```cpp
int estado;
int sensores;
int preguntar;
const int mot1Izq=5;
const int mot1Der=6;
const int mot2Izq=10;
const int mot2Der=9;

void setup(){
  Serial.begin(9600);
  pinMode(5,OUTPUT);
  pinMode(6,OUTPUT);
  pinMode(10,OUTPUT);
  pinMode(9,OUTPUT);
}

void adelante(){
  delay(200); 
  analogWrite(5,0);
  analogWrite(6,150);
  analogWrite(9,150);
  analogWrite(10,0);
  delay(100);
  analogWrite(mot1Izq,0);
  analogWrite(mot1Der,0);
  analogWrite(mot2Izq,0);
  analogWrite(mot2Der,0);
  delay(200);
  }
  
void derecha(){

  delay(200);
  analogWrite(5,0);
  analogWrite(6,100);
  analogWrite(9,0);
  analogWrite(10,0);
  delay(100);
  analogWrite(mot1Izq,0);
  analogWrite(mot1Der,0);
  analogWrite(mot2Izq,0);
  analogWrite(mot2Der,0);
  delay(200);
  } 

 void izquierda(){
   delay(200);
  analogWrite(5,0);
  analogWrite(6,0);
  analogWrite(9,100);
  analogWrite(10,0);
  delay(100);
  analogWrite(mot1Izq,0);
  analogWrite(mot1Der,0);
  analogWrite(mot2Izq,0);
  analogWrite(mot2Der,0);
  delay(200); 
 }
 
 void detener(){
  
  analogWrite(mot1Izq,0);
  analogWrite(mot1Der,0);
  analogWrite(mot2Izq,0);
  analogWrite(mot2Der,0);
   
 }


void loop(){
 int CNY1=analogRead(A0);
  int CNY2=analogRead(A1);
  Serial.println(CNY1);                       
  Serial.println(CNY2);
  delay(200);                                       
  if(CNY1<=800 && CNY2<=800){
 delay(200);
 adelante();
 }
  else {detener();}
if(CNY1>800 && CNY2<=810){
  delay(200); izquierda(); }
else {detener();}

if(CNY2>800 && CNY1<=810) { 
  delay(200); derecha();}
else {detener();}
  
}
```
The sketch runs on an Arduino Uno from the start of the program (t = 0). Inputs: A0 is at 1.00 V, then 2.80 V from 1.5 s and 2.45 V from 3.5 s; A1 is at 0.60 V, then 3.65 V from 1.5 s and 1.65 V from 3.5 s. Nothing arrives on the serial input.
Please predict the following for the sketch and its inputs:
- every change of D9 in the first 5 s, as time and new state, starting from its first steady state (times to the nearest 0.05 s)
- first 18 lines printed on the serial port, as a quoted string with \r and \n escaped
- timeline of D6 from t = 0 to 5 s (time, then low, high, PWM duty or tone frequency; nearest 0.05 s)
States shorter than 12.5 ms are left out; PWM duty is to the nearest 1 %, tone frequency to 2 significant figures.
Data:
0 s low; 0.6 s PWM 59 %; 0.7 s low; 1.5 s PWM 59 %; 1.6 s low; 2.4 s PWM 59 %; 2.5 s low; 3.3 s PWM 59 %; 3.4 s low; 4.2 s PWM 59 %; 4.3 s low
"204\r\n122\r\n204\r\n122\r\n573\r\n747\r\n573\r\n747\r\n501\r\n337\r\n501\r\n337\r\n501\r\n337\r\n501\r\n337\r\n501\r\n337\r\n"
0 s low; 0.6 s PWM 59 %; 0.7 s low; 1.5 s PWM 59 %; 1.6 s low; 2.4 s PWM 59 %; 2.5 s low; 3.3 s PWM 59 %; 3.4 s low; 4.2 s PWM 59 %; 4.3 s low
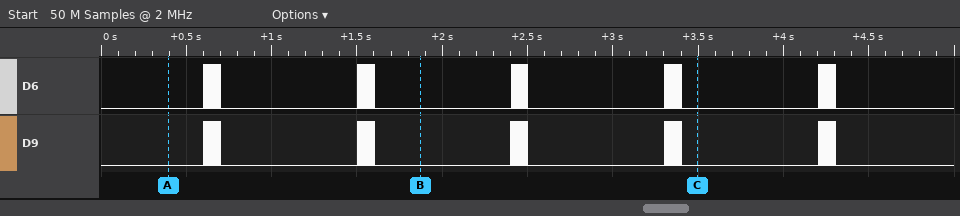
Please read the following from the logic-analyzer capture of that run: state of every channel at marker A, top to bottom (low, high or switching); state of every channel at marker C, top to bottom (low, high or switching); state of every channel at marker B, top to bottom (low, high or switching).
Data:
D6 low, D9 low
D6 low, D9 low
D6 low, D9 low
